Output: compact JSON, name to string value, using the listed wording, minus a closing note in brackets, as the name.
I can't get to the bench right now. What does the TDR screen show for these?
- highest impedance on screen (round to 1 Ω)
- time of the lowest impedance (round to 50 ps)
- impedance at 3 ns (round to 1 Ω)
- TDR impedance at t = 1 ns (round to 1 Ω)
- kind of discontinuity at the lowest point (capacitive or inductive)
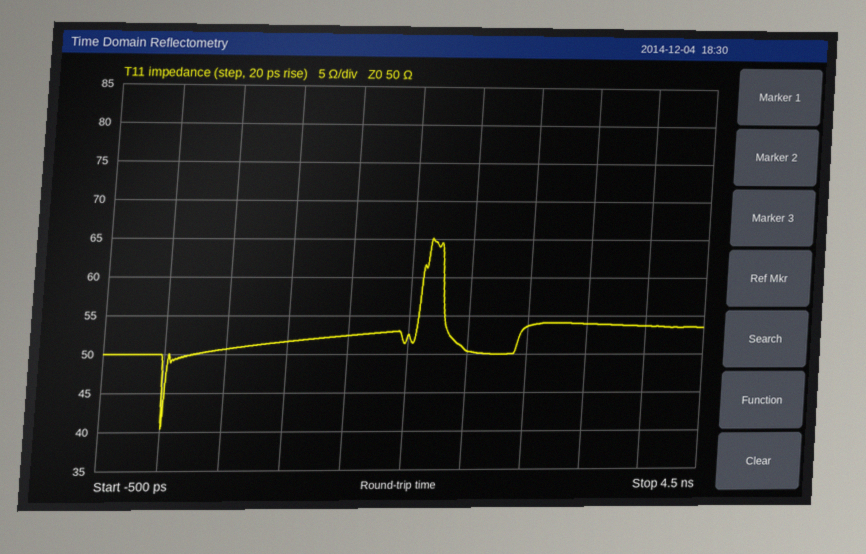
{"highest impedance on screen": "65 Ω", "time of the lowest impedance": "0 ps", "impedance at 3 ns": "54 Ω", "TDR impedance at t = 1 ns": "52 Ω", "kind of discontinuity at the lowest point": "capacitive"}
